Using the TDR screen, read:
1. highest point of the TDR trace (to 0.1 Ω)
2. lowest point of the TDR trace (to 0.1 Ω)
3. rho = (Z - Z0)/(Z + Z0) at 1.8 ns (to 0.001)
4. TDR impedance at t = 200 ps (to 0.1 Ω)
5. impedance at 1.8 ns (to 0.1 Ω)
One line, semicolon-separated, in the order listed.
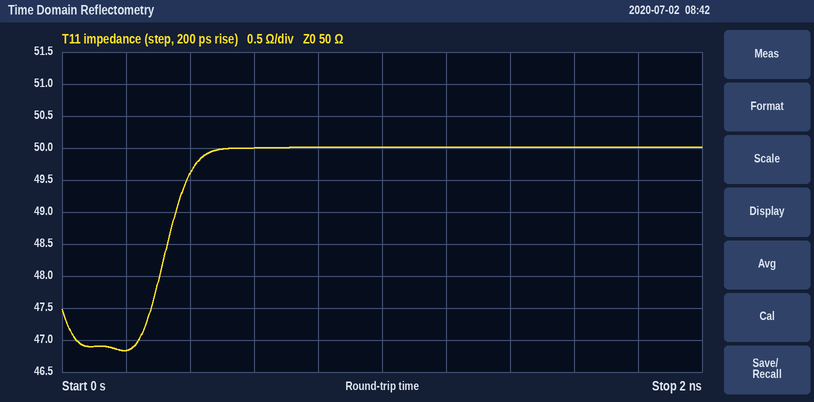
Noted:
50.0 Ω; 46.8 Ω; 0.000; 46.8 Ω; 50.0 Ω
